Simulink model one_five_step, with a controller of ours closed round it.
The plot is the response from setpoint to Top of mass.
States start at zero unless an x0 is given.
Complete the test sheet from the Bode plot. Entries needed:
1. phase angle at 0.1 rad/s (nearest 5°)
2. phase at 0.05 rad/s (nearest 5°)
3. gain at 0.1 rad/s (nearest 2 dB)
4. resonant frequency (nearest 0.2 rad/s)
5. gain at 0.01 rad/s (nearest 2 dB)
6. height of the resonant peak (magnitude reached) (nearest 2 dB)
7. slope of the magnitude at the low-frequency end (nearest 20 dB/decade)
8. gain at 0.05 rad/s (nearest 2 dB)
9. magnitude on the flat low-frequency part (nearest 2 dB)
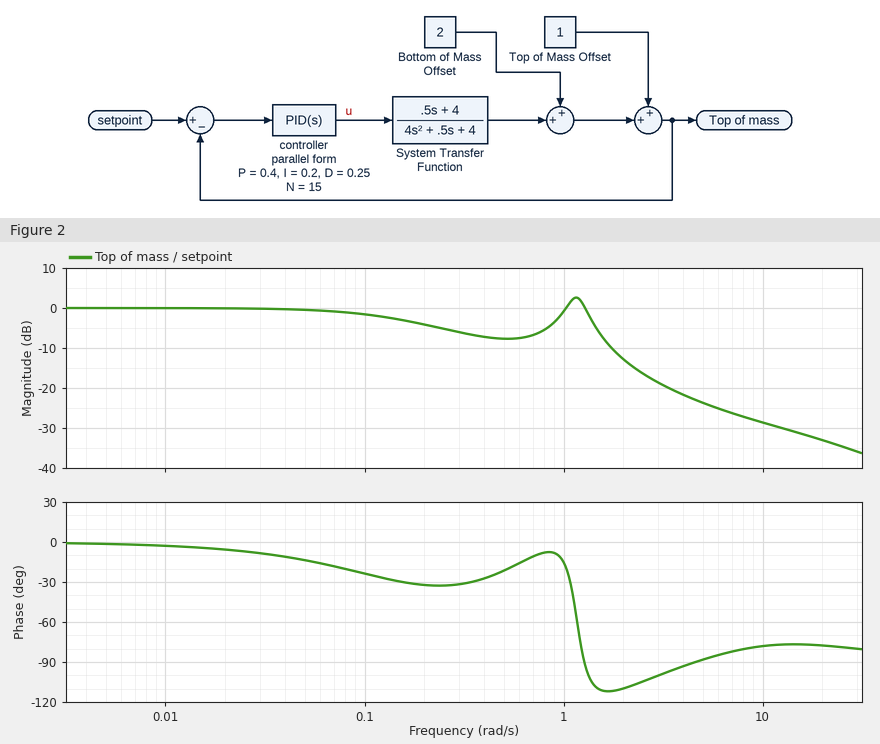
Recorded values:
-25°
-15°
-2 dB
1.2 rad/s
0 dB
2 dB
0 dB/decade
0 dB
0 dB
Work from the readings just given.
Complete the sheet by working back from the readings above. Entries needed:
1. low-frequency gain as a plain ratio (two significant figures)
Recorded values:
1.0
